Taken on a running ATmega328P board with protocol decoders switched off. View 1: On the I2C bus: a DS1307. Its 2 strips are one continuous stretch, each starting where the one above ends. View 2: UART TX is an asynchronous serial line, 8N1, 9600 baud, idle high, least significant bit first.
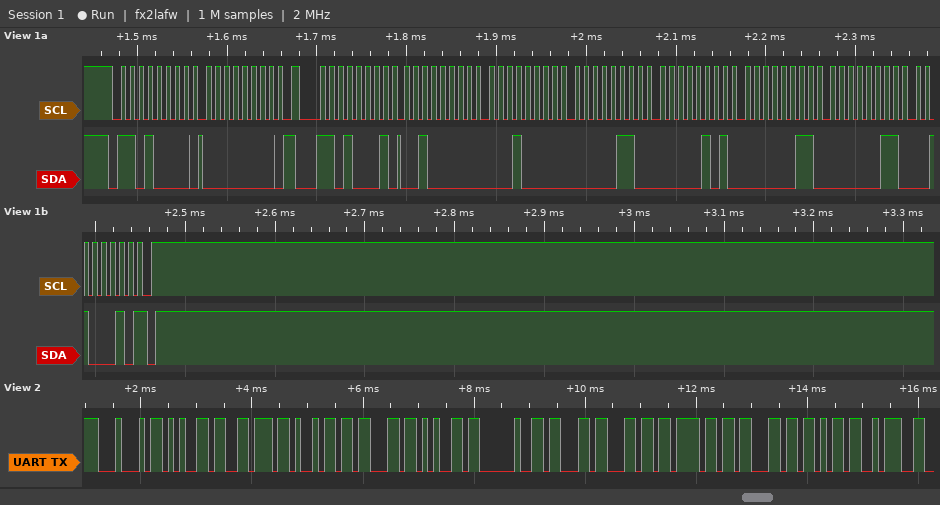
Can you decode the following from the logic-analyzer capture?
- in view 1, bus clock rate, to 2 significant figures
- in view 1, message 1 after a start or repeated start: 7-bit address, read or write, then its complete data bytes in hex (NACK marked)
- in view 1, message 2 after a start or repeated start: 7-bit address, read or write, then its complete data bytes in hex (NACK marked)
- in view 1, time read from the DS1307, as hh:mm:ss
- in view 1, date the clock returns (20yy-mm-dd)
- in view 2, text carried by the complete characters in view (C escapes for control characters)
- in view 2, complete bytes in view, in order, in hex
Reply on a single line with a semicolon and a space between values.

100 kHz; 0x68 write: 00; 0x68 read: 20 10 06 05 03 03 22 NACK; 06:10:20; 2022-03-03; "Device clock:"; 44 65 76 69 63 65 20 63 6C 6F 63 6B 3A
